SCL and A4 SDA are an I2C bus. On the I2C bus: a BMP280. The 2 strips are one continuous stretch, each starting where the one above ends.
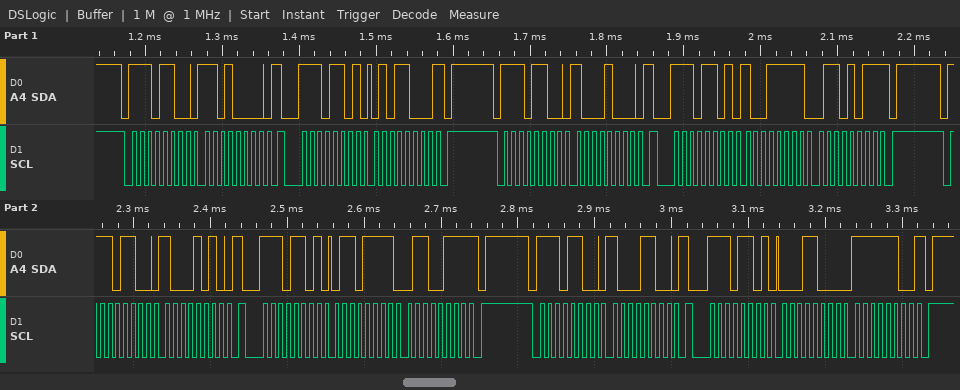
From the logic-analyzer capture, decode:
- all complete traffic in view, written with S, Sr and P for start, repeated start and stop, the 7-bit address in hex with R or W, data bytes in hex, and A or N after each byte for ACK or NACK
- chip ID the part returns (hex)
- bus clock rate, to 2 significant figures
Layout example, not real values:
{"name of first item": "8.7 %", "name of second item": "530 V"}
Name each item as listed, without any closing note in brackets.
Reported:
{"all complete traffic in view, written with S, Sr and P for start, repeated start and stop, the 7-bit address in hex with R or W, data bytes in hex, and A or N after each byte for ACK or NACK": "S 76W A D0 A Sr 76R A 58 N P S 76W A 88 A Sr 76R A 9F A 6B N P S 76W A 8A A Sr 76R A 6F A 67 N P S 76W A 8C A Sr 76R A 18 A FC N P", "chip ID the part returns": "0x58", "bus clock rate, to 2 significant figures": "100 kHz"}
